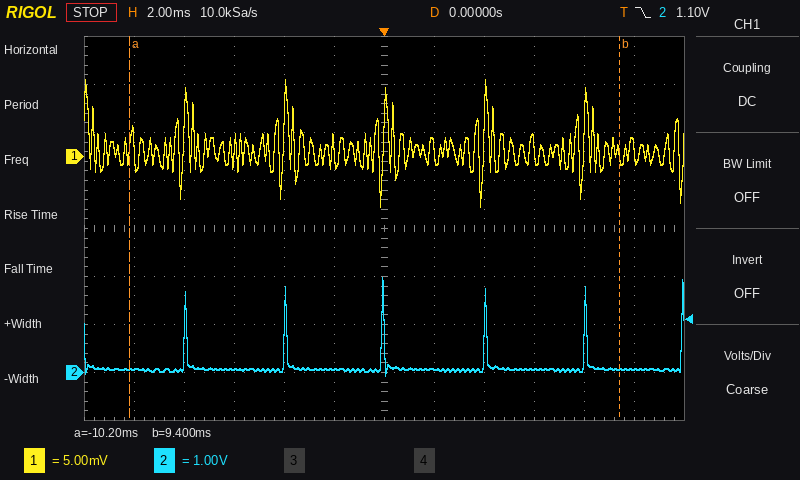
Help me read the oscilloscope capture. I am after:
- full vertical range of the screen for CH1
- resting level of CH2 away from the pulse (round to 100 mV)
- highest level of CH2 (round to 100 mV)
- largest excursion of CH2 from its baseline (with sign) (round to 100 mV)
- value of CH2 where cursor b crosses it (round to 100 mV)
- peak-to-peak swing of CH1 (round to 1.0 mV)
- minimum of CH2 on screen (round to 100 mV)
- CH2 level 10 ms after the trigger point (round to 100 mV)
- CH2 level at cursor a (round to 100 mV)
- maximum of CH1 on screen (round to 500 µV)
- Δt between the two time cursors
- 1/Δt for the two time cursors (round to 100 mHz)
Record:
40 mV
100 mV
2.0 V
+1.9 V
100 mV
13.0 mV
-100 mV
100 mV
100 mV
8.0 mV
19.6 ms
51.0 Hz
